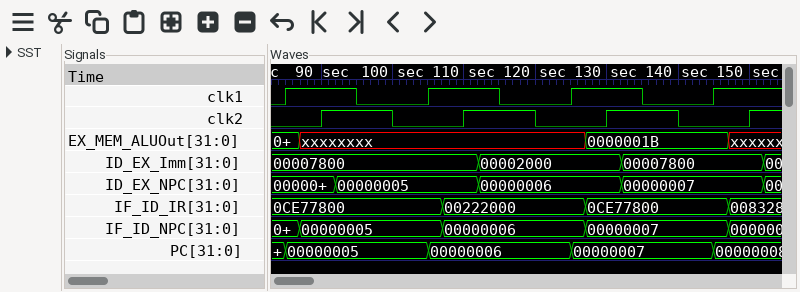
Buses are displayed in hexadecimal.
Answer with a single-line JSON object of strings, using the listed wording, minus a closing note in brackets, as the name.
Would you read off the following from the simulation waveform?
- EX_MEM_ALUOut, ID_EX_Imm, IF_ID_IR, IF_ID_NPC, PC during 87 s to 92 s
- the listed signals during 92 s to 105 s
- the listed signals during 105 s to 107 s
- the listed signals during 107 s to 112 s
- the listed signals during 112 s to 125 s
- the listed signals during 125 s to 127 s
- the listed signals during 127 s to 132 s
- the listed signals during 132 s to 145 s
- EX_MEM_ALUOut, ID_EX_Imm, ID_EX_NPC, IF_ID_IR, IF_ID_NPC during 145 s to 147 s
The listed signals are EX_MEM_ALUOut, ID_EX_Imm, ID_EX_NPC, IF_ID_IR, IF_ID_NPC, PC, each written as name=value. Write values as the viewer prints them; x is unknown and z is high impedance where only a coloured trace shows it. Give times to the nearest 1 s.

{"EX_MEM_ALUOut, ID_EX_Imm, IF_ID_IR, IF_ID_NPC, PC during 87 s to 92 s": "EX_MEM_ALUOut=xxxxxxxx, ID_EX_Imm=00007800, IF_ID_IR=0CE77800, IF_ID_NPC=00000005, PC=00000005", "the listed signals during 92 s to 105 s": "EX_MEM_ALUOut=xxxxxxxx, ID_EX_Imm=00007800, ID_EX_NPC=00000005, IF_ID_IR=0CE77800, IF_ID_NPC=00000005, PC=00000005", "the listed signals during 105 s to 107 s": "EX_MEM_ALUOut=xxxxxxxx, ID_EX_Imm=00007800, ID_EX_NPC=00000005, IF_ID_IR=0CE77800, IF_ID_NPC=00000005, PC=00000006", "the listed signals during 107 s to 112 s": "EX_MEM_ALUOut=xxxxxxxx, ID_EX_Imm=00007800, ID_EX_NPC=00000005, IF_ID_IR=00222000, IF_ID_NPC=00000006, PC=00000006", "the listed signals during 112 s to 125 s": "EX_MEM_ALUOut=xxxxxxxx, ID_EX_Imm=00002000, ID_EX_NPC=00000006, IF_ID_IR=00222000, IF_ID_NPC=00000006, PC=00000006", "the listed signals during 125 s to 127 s": "EX_MEM_ALUOut=xxxxxxxx, ID_EX_Imm=00002000, ID_EX_NPC=00000006, IF_ID_IR=00222000, IF_ID_NPC=00000006, PC=00000007", "the listed signals during 127 s to 132 s": "EX_MEM_ALUOut=0000001B, ID_EX_Imm=00002000, ID_EX_NPC=00000006, IF_ID_IR=0CE77800, IF_ID_NPC=00000007, PC=00000007", "the listed signals during 132 s to 145 s": "EX_MEM_ALUOut=0000001B, ID_EX_Imm=00007800, ID_EX_NPC=00000007, IF_ID_IR=0CE77800, IF_ID_NPC=00000007, PC=00000007", "EX_MEM_ALUOut, ID_EX_Imm, ID_EX_NPC, IF_ID_IR, IF_ID_NPC during 145 s to 147 s": "EX_MEM_ALUOut=0000001B, ID_EX_Imm=00007800, ID_EX_NPC=00000007, IF_ID_IR=0CE77800, IF_ID_NPC=00000007"}
